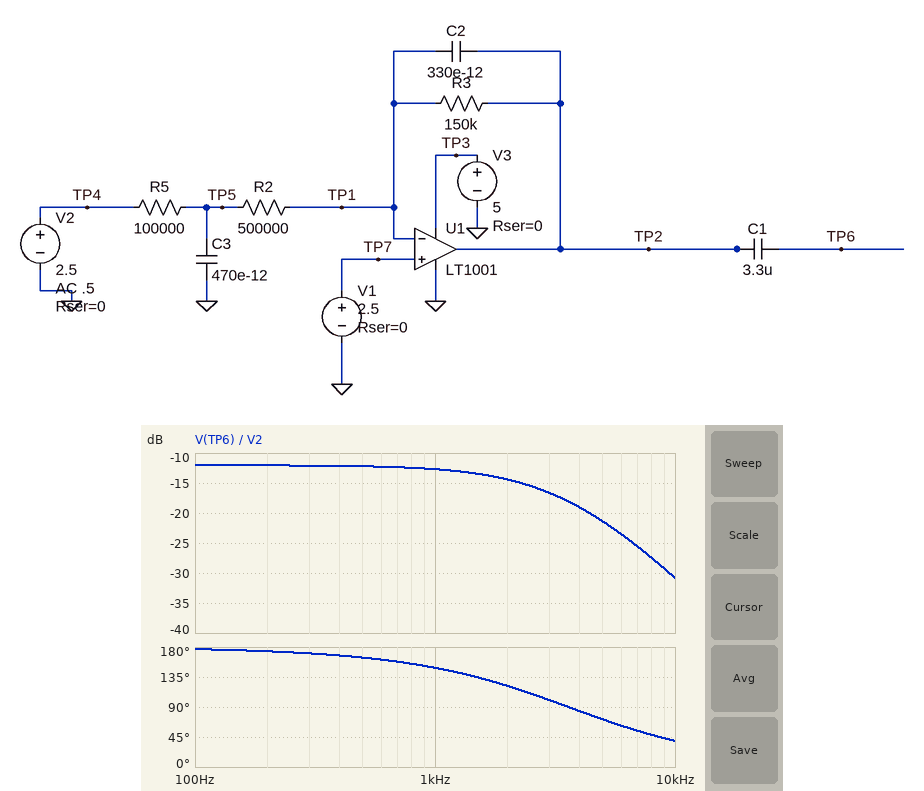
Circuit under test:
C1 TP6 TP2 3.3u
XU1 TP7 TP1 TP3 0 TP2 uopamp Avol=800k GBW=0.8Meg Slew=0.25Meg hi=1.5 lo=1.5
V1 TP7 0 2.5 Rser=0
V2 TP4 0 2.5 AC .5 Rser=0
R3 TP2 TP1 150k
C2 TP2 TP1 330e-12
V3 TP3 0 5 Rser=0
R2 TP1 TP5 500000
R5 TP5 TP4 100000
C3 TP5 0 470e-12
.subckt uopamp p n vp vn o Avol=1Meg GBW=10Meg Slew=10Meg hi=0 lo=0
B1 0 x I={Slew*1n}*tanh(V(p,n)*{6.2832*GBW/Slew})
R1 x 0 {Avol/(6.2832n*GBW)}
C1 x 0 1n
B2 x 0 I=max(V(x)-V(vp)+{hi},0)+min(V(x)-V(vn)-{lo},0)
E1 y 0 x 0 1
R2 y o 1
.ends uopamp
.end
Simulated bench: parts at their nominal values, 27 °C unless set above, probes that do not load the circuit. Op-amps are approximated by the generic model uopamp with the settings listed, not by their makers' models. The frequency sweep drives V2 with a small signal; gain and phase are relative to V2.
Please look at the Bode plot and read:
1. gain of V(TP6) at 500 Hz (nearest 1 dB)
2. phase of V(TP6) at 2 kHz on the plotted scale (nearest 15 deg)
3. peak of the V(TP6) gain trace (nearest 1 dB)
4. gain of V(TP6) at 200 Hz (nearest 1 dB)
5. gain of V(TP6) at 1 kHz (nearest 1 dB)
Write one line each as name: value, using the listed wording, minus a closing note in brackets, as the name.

gain of V(TP6) at 500 Hz: -12 dB
phase of V(TP6) at 2 kHz on the plotted scale: 120 deg
peak of the V(TP6) gain trace: -12 dB
gain of V(TP6) at 200 Hz: -12 dB
gain of V(TP6) at 1 kHz: -13 dB
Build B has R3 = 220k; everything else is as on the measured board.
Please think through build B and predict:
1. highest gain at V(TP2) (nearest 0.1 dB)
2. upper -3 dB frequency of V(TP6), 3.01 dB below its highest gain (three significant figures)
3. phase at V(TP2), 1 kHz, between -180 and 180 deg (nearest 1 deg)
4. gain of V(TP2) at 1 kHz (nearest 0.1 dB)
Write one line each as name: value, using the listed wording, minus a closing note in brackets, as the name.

highest gain at V(TP2): -8.7 dB
upper -3 dB frequency of V(TP6), 3.01 dB below its highest gain: 1.80 kHz
phase at V(TP2), 1 kHz, between -180 and 180 deg: 142 deg
gain of V(TP2) at 1 kHz: -9.8 dB
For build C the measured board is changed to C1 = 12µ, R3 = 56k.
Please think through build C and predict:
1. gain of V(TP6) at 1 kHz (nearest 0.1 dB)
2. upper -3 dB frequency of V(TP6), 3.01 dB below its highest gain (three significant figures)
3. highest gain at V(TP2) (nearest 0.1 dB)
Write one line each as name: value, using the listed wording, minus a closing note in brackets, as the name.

gain of V(TP6) at 1 kHz: -20.9 dB
upper -3 dB frequency of V(TP6), 3.01 dB below its highest gain: 3.45 kHz
highest gain at V(TP2): -20.6 dB
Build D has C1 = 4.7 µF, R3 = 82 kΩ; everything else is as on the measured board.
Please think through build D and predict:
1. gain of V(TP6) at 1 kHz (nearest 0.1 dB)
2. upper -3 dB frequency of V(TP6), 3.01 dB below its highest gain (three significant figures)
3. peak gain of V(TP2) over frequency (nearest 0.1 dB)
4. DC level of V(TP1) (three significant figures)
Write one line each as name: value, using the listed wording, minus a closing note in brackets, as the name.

gain of V(TP6) at 1 kHz: -17.7 dB
upper -3 dB frequency of V(TP6), 3.01 dB below its highest gain: 3.07 kHz
peak gain of V(TP2) over frequency: -17.3 dB
DC level of V(TP1): 2.50 V
